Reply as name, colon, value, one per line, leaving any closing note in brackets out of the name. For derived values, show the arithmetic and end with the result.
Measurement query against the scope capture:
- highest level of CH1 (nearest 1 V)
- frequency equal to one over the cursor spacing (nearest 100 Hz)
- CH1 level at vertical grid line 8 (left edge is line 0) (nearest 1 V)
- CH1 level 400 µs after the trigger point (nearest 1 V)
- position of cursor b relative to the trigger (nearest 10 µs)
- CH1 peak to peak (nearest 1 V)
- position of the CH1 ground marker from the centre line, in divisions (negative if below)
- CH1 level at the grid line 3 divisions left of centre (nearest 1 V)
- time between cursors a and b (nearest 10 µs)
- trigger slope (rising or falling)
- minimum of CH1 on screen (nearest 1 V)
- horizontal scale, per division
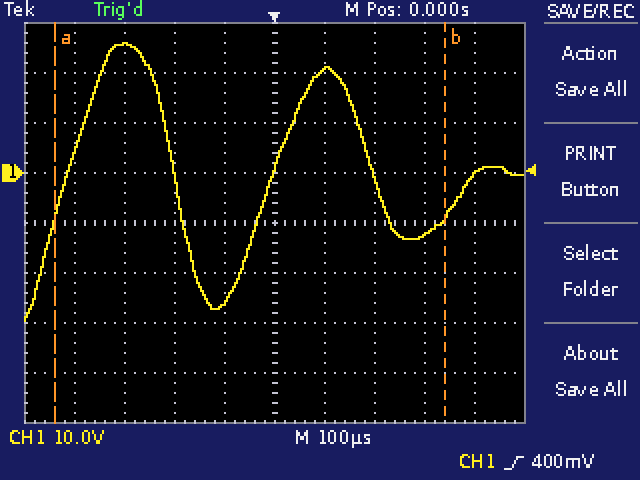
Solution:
highest level of CH1: 26 V
frequency equal to one over the cursor spacing: 1 / 780 µs ≈ 1.3 kHz
CH1 level at vertical grid line 8 (left edge is line 0): -12 V
CH1 level 400 µs after the trigger point: 0 V
position of cursor b relative to the trigger: +340 µs
CH1 peak to peak: 26 V − (-30 V) = 56 V
position of the CH1 ground marker from the centre line, in divisions: +1.0 div
CH1 level at the grid line 3 divisions left of centre: 26 V
time between cursors a and b: 780 µs
trigger slope: rising
minimum of CH1 on screen: -30 V
horizontal scale, per division: 100 µs
